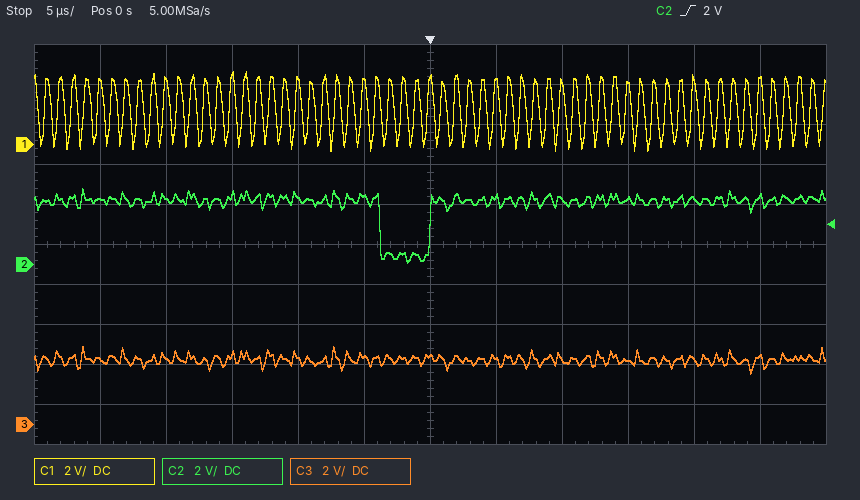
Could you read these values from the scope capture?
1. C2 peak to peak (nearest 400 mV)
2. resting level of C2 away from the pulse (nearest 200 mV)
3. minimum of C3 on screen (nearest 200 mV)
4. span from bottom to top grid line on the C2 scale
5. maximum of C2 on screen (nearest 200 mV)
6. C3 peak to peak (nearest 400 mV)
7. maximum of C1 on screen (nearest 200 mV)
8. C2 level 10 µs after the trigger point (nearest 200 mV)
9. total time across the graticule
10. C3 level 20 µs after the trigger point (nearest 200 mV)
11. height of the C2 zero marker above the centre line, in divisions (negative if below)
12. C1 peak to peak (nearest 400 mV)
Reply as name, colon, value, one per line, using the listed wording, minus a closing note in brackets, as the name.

C2 peak to peak: 3.6 V
resting level of C2 away from the pulse: 3.2 V
minimum of C3 on screen: 2.6 V
span from bottom to top grid line on the C2 scale: 20 V
maximum of C2 on screen: 3.8 V
C3 peak to peak: 1.2 V
maximum of C1 on screen: 3.6 V
C2 level 10 µs after the trigger point: 3.2 V
total time across the graticule: 60 µs
C3 level 20 µs after the trigger point: 3.2 V
height of the C2 zero marker above the centre line, in divisions: -0.5 div
C1 peak to peak: 4.0 V
